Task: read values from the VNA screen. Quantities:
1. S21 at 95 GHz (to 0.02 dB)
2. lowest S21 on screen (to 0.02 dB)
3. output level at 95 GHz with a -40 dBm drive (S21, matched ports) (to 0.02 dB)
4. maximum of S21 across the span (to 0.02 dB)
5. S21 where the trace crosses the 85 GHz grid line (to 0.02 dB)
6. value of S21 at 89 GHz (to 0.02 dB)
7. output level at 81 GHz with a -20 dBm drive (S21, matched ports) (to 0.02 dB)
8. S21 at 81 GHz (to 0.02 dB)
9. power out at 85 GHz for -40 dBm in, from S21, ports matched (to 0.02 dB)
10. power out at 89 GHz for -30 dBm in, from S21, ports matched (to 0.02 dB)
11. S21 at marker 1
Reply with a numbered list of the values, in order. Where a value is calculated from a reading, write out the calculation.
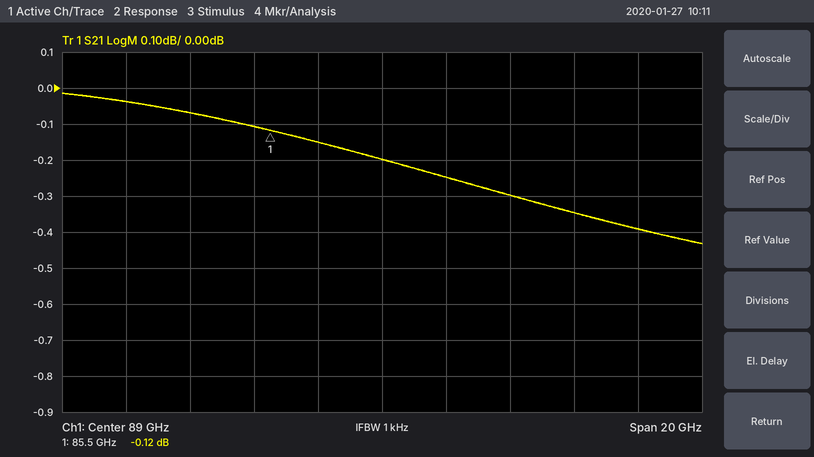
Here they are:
1. -0.34 dB
2. -0.44 dB
3. -40 dBm + (-0.34 dB) = -40.34 dBm
4. -0.02 dB
5. -0.10 dB
6. -0.20 dB
7. -20 dBm + (-0.04 dB) = -20.04 dBm
8. -0.04 dB
9. -40 dBm + (-0.10 dB) = -40.10 dBm
10. -30 dBm + (-0.20 dB) = -30.20 dBm
11. -0.12 dB
